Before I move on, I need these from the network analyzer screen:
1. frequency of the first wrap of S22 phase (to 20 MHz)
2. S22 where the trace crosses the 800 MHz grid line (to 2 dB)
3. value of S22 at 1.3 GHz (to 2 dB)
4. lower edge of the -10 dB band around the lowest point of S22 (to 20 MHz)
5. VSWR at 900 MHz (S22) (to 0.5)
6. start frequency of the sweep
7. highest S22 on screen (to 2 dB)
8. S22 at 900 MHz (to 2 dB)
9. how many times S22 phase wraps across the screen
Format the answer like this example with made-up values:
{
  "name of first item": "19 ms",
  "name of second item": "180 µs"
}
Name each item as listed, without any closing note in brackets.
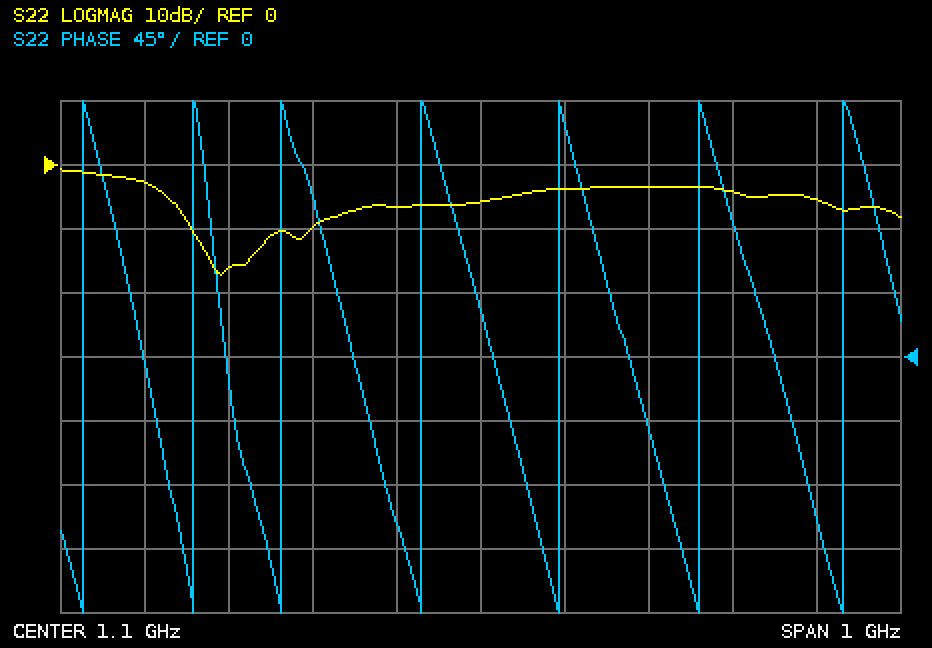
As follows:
{
  "frequency of the first wrap of S22 phase": "620 MHz",
  "S22 where the trace crosses the 800 MHz grid line": "-16 dB",
  "value of S22 at 1.3 GHz": "-4 dB",
  "lower edge of the -10 dB band around the lowest point of S22": "760 MHz",
  "VSWR at 900 MHz (S22)": "2.0",
  "start frequency of the sweep": "600 MHz",
  "highest S22 on screen": "0 dB",
  "S22 at 900 MHz": "-10 dB",
  "how many times S22 phase wraps across the screen": "7"
}
